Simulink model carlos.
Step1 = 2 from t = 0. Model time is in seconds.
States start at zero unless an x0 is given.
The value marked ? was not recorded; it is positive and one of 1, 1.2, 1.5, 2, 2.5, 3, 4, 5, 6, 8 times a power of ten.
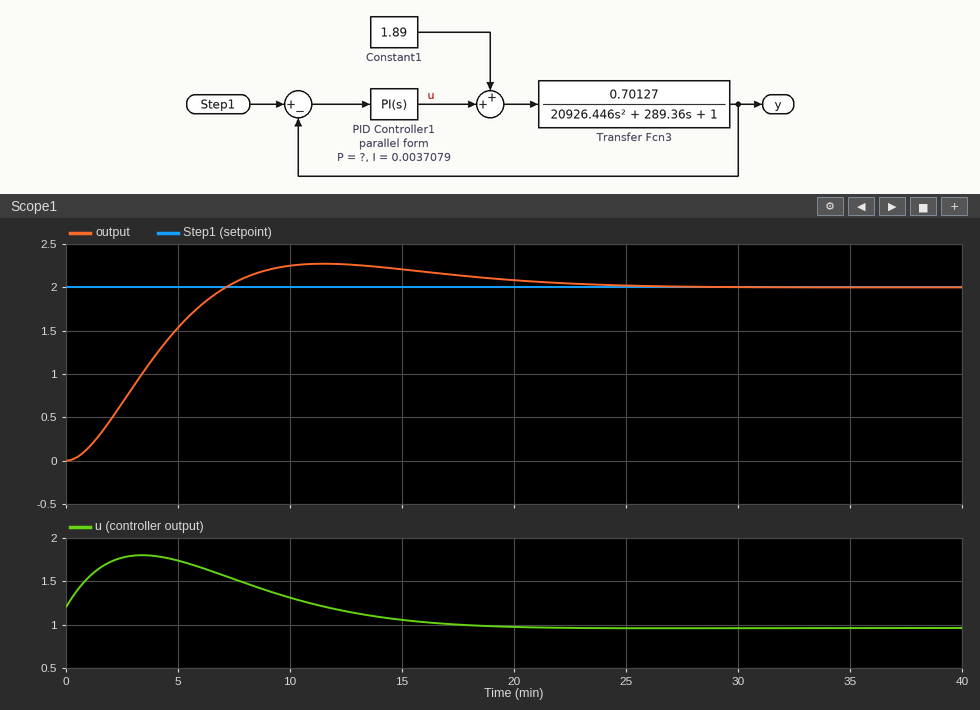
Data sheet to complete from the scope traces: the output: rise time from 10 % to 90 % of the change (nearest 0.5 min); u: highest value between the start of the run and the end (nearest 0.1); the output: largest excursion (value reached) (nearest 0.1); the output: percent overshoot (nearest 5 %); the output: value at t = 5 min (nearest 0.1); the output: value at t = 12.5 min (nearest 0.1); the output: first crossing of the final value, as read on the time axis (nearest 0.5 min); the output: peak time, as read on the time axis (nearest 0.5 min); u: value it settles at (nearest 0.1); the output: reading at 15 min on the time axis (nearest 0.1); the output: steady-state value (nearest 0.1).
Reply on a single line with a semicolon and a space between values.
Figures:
5.0 min; 1.8; 2.3; 15 %; 1.5; 2.3; 7.0 min; 11.5 min; 1.0; 2.2; 2.0
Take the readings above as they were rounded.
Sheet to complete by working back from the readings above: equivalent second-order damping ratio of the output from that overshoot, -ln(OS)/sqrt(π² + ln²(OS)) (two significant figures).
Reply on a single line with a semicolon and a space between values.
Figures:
0.52
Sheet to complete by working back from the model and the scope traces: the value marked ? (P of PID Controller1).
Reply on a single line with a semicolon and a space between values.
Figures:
0.6
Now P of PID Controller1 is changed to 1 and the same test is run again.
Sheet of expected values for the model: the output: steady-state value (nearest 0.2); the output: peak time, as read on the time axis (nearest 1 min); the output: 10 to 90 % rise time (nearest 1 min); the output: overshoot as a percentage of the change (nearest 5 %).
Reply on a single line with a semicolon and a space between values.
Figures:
2.0; 10 min; 4 min; 10 %
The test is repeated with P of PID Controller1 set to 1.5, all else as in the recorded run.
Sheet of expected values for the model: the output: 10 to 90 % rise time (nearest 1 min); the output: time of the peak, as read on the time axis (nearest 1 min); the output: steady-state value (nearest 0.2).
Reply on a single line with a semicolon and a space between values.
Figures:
4 min; 8 min; 2.0
